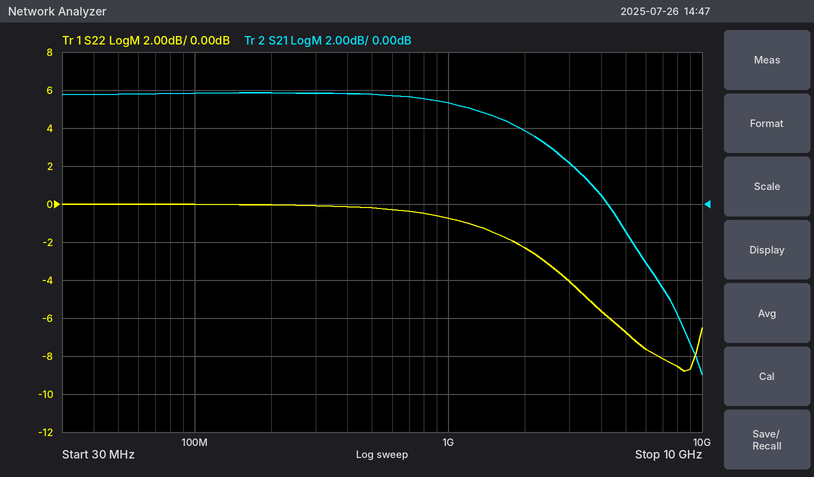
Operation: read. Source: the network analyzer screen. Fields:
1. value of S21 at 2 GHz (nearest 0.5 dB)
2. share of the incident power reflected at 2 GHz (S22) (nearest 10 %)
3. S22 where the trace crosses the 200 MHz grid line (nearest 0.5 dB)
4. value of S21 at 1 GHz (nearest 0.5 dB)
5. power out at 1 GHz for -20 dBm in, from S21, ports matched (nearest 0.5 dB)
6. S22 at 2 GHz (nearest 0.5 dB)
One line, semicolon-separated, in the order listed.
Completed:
4.0 dB; 60 %; 0.0 dB; 5.5 dB; -14.5 dBm; -2.5 dB
